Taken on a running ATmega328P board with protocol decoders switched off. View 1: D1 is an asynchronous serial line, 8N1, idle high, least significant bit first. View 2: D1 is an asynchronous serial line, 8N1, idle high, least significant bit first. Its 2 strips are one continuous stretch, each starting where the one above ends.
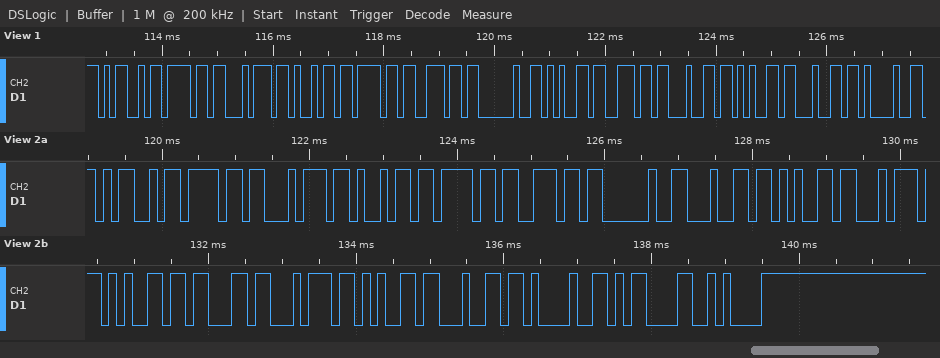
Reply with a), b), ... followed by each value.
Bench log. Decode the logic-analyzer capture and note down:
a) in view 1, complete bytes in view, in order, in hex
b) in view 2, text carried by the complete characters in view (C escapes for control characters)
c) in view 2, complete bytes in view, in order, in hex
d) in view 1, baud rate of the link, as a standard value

a) 0x4D 0x6F 0x74 0x69 0x6F 0x6E 0x20 0x65 0x6E 0x64 0x65 0x64 0x21
b) "Motion detected!\r\n"
c) 4D 6F 74 69 6F 6E 20 64 65 74 65 63 74 65 64 21 0D 0A
d) 9600 baud
